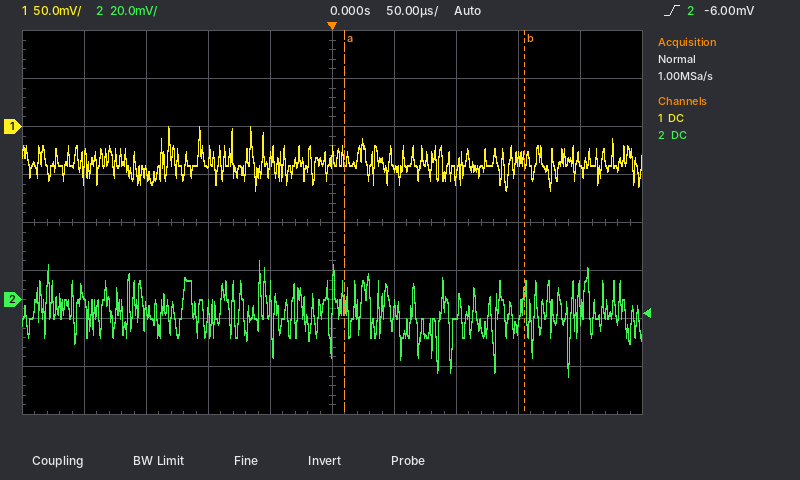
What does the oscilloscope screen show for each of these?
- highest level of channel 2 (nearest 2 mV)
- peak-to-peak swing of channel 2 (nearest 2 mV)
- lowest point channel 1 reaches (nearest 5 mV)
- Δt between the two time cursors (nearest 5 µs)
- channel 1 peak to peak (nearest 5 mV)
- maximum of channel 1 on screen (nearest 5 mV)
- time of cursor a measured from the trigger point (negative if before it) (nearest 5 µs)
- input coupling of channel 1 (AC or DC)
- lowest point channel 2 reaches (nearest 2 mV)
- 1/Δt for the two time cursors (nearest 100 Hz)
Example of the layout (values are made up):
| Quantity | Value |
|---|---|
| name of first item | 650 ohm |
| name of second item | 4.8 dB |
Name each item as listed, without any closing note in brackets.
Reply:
| Quantity | Value |
|---|---|
| highest level of channel 2 | 16 mV |
| peak-to-peak swing of channel 2 | 48 mV |
| lowest point channel 1 reaches | -65 mV |
| Δt between the two time cursors | 145 µs |
| channel 1 peak to peak | 65 mV |
| maximum of channel 1 on screen | 0 mV |
| time of cursor a measured from the trigger point (negative if before it) | +10 µs |
| input coupling of channel 1 | DC |
| lowest point channel 2 reaches | -32 mV |
| 1/Δt for the two time cursors | 6.9 kHz |
